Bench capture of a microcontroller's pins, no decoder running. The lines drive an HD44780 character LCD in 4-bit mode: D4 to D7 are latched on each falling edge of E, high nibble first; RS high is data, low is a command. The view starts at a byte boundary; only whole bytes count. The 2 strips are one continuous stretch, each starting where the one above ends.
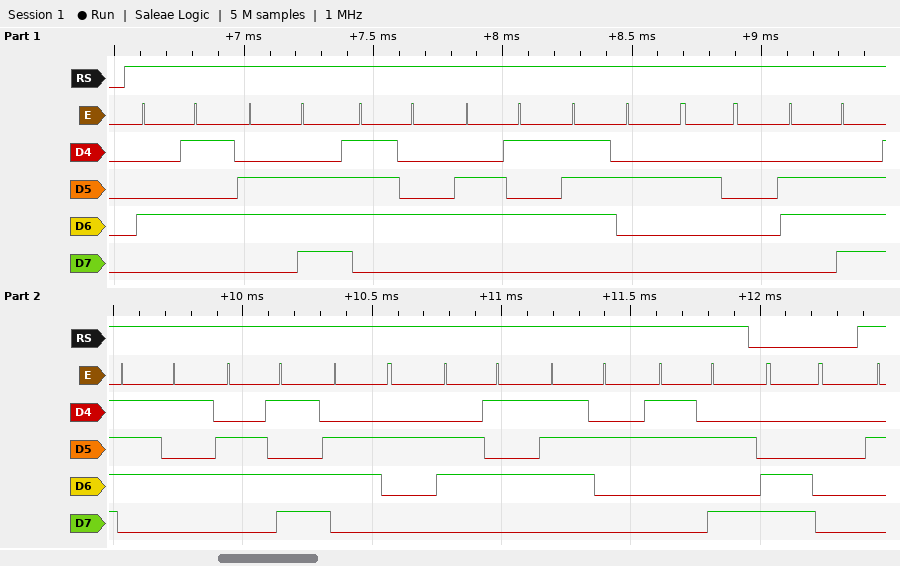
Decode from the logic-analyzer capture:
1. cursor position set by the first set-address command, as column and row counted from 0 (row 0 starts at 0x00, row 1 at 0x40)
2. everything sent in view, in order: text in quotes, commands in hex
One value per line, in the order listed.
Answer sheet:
column 0, row 1
"Enter number:" 0xC0
